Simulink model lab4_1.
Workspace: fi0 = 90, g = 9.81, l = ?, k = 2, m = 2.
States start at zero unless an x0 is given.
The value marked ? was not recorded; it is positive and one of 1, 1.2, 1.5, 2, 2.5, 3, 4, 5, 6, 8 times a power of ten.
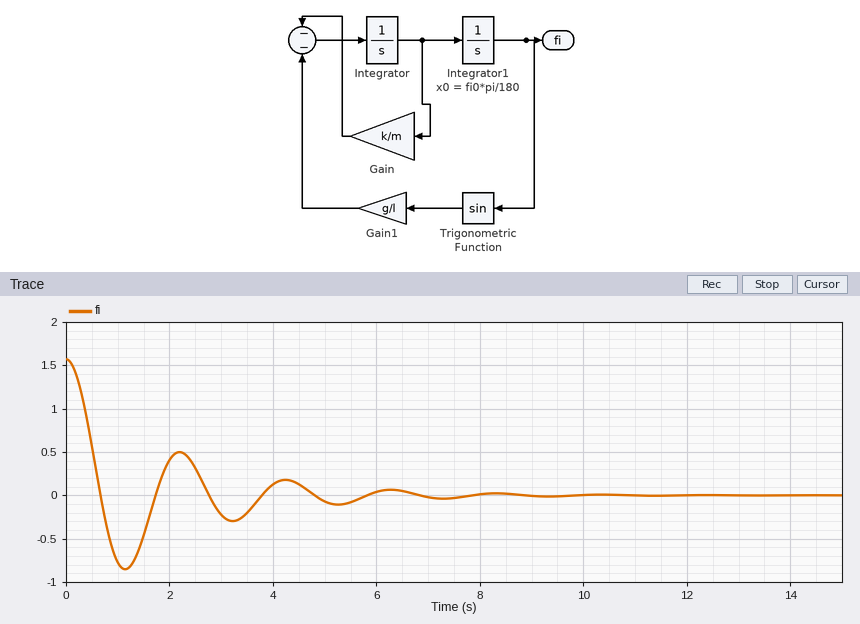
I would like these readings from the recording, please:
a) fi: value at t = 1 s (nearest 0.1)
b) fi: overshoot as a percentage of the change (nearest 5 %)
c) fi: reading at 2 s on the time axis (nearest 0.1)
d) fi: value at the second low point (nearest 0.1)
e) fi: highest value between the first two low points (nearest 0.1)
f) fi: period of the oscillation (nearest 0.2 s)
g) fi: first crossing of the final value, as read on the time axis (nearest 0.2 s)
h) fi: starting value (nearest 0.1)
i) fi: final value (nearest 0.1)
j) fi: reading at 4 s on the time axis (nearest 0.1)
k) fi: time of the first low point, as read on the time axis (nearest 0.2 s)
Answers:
-0.8
55 %
0.4
-0.3
0.5
2.0 s
0.6 s
1.6
0.0
0.1
1.2 s
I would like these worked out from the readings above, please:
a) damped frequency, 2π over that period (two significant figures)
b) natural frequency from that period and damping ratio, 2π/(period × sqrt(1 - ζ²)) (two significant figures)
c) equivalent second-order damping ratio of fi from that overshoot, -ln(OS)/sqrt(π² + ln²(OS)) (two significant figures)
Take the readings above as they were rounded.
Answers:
3.1 rad/s
3.2 rad/s
0.19
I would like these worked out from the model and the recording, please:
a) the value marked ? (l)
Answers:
1
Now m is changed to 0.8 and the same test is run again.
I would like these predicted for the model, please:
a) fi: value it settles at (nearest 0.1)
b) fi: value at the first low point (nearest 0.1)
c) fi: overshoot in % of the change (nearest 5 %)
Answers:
0.0
-0.3
20 %
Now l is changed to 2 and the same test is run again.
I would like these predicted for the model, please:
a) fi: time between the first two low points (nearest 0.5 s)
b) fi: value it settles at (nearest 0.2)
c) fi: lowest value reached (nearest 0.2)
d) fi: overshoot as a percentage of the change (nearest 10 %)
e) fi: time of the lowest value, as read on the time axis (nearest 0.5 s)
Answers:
3.0 s
0.0
-0.6
40 %
1.5 s
